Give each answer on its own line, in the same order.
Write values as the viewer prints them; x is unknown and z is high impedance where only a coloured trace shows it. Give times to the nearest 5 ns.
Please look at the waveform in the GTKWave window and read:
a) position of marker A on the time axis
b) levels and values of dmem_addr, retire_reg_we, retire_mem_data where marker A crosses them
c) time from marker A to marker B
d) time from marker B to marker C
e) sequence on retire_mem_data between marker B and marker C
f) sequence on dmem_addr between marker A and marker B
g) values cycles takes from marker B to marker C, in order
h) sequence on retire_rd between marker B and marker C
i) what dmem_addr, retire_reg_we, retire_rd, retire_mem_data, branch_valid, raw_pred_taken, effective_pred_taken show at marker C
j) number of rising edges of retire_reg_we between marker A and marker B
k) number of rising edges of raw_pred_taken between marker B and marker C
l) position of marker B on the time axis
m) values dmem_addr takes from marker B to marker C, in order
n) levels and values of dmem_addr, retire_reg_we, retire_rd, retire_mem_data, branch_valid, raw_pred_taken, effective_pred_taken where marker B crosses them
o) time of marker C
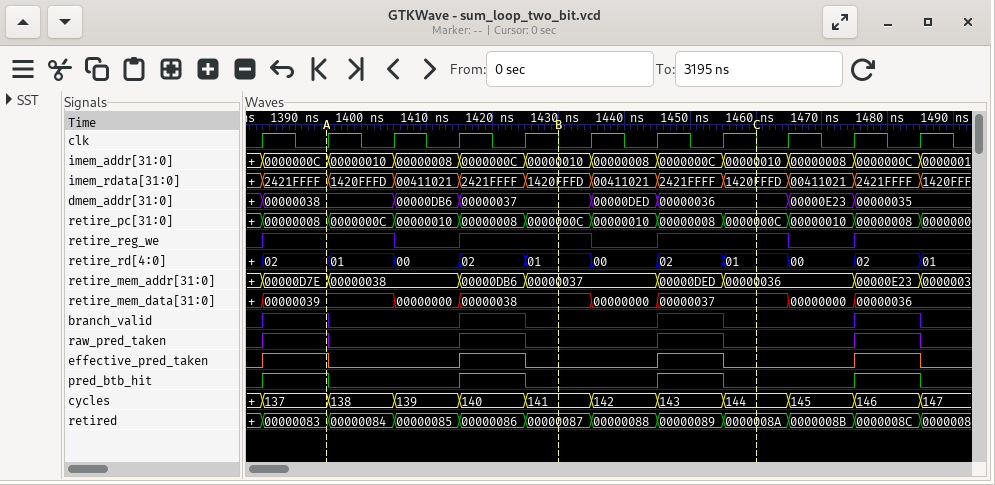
1395 ns
dmem_addr=00000038, retire_reg_we=1, retire_mem_data=00000039
35 ns
30 ns
00000038, 00000000, 00000037
00000038, 00000DB6, 00000037
141, 142, 143, 144
01, 00, 02, 01
dmem_addr=00000036, retire_reg_we=1, retire_rd=01, retire_mem_data=00000037, branch_valid=0, raw_pred_taken=0, effective_pred_taken=0
1
1
1430 ns
00000037, 00000DED, 00000036
dmem_addr=00000037, retire_reg_we=1, retire_rd=01, retire_mem_data=00000038, branch_valid=0, raw_pred_taken=0, effective_pred_taken=0
1460 ns
